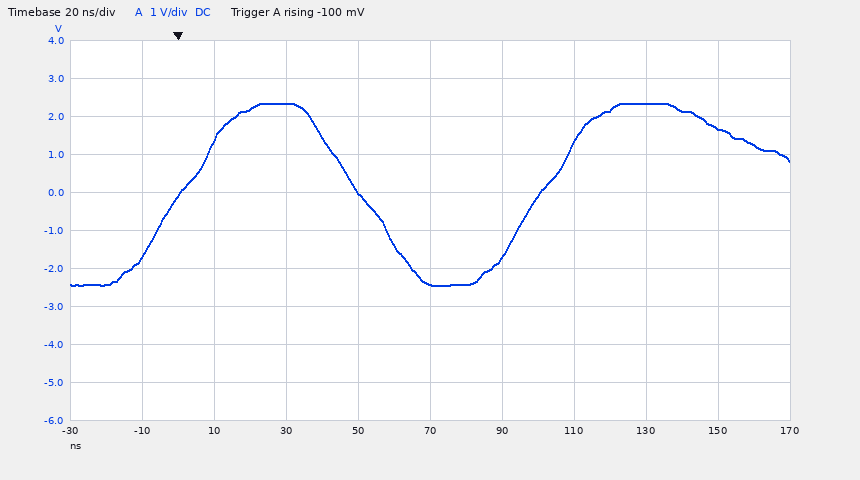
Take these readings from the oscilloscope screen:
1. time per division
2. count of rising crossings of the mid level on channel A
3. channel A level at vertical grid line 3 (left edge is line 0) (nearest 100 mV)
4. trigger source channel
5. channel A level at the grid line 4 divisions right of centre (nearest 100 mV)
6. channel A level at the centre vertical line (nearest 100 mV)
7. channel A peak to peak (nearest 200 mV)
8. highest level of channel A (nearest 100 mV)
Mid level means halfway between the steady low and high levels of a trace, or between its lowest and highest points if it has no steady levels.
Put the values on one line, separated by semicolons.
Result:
20 ns; 2; 2.3 V; channel A; 1.7 V; -2.4 V; 4.8 V; 2.3 V
